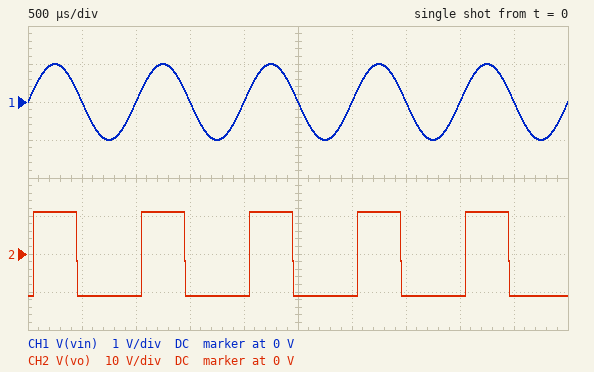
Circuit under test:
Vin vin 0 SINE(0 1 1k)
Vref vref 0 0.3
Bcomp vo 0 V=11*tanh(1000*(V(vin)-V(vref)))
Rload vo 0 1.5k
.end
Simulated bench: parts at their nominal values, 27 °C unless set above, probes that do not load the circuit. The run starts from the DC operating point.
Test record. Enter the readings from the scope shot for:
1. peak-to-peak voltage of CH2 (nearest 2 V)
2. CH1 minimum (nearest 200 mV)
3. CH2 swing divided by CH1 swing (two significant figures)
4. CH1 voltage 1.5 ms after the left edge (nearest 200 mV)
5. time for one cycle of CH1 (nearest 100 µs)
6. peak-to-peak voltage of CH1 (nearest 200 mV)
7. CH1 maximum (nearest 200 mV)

22 V
-1.0 V
11
0 V
1.0 ms
2.0 V
1.0 V
